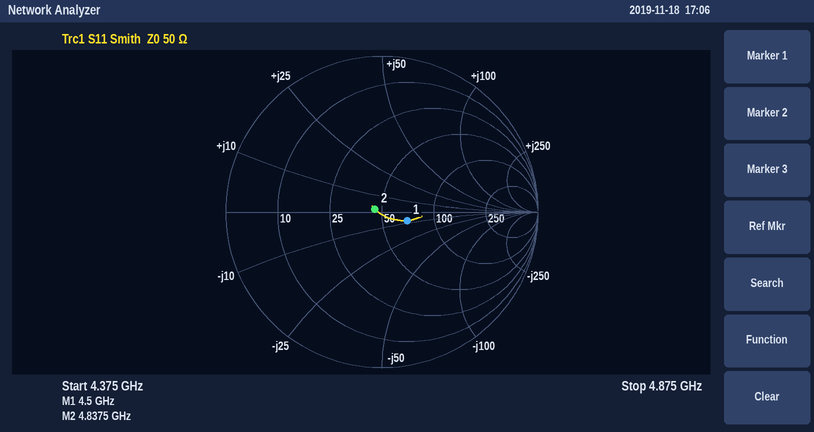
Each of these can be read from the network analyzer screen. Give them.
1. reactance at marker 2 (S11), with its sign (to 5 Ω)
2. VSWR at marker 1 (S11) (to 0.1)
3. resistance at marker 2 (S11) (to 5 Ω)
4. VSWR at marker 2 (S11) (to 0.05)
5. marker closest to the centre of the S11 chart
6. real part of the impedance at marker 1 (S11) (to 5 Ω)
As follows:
0 Ω
1.4
45 Ω
1.10
marker 2
70 Ω
